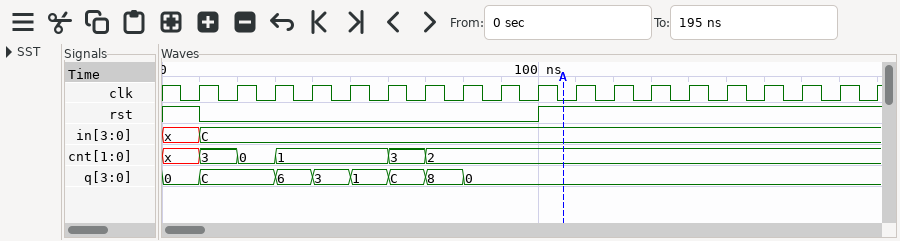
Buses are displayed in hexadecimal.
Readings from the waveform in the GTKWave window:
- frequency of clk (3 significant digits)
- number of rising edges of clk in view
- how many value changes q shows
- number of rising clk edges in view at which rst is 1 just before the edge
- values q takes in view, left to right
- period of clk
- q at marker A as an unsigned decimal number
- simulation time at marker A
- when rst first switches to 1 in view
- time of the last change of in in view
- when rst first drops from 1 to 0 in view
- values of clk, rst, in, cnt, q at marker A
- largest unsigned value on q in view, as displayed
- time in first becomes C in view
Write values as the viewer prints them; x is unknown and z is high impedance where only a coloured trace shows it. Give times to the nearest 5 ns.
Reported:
100 MHz
19
7
10
0, C, 6, 3, 1, C, 8, 0
10 ns
0
105 ns
100 ns
10 ns
10 ns
clk=0, rst=1, in=C, cnt=2, q=0
C
10 ns
